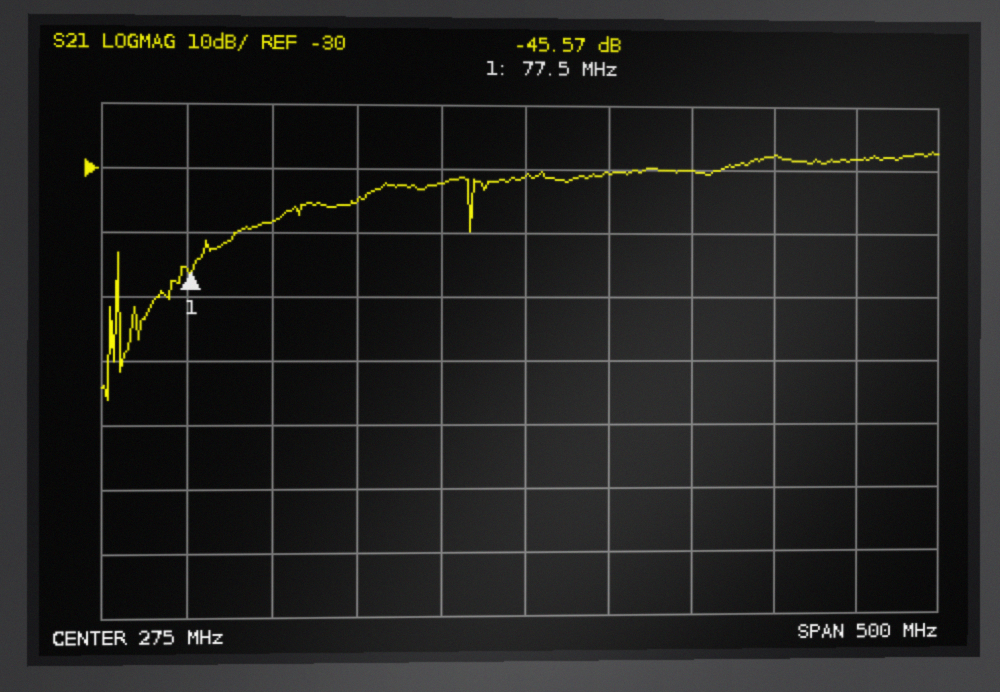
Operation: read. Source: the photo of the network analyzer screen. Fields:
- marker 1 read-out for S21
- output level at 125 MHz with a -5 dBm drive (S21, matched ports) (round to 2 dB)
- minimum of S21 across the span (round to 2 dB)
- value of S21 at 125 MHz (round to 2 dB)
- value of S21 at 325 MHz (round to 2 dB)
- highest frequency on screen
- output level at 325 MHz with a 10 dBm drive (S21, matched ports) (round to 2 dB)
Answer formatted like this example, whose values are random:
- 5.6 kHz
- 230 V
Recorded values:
- -45.57 dB
- -44 dBm
- -66 dB
- -38 dB
- -30 dB
- 525 MHz
- -20 dBm
